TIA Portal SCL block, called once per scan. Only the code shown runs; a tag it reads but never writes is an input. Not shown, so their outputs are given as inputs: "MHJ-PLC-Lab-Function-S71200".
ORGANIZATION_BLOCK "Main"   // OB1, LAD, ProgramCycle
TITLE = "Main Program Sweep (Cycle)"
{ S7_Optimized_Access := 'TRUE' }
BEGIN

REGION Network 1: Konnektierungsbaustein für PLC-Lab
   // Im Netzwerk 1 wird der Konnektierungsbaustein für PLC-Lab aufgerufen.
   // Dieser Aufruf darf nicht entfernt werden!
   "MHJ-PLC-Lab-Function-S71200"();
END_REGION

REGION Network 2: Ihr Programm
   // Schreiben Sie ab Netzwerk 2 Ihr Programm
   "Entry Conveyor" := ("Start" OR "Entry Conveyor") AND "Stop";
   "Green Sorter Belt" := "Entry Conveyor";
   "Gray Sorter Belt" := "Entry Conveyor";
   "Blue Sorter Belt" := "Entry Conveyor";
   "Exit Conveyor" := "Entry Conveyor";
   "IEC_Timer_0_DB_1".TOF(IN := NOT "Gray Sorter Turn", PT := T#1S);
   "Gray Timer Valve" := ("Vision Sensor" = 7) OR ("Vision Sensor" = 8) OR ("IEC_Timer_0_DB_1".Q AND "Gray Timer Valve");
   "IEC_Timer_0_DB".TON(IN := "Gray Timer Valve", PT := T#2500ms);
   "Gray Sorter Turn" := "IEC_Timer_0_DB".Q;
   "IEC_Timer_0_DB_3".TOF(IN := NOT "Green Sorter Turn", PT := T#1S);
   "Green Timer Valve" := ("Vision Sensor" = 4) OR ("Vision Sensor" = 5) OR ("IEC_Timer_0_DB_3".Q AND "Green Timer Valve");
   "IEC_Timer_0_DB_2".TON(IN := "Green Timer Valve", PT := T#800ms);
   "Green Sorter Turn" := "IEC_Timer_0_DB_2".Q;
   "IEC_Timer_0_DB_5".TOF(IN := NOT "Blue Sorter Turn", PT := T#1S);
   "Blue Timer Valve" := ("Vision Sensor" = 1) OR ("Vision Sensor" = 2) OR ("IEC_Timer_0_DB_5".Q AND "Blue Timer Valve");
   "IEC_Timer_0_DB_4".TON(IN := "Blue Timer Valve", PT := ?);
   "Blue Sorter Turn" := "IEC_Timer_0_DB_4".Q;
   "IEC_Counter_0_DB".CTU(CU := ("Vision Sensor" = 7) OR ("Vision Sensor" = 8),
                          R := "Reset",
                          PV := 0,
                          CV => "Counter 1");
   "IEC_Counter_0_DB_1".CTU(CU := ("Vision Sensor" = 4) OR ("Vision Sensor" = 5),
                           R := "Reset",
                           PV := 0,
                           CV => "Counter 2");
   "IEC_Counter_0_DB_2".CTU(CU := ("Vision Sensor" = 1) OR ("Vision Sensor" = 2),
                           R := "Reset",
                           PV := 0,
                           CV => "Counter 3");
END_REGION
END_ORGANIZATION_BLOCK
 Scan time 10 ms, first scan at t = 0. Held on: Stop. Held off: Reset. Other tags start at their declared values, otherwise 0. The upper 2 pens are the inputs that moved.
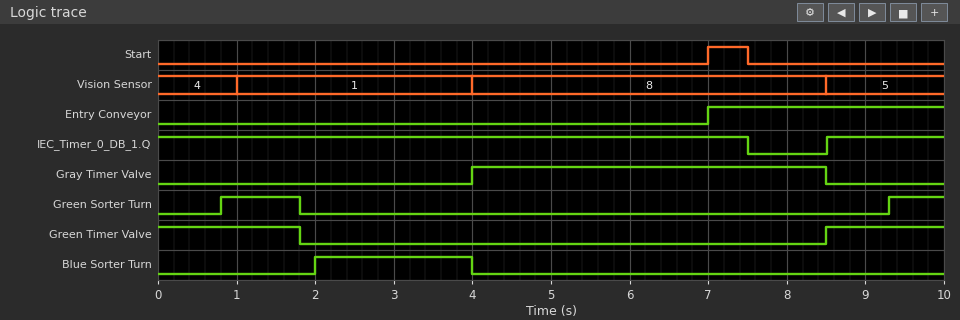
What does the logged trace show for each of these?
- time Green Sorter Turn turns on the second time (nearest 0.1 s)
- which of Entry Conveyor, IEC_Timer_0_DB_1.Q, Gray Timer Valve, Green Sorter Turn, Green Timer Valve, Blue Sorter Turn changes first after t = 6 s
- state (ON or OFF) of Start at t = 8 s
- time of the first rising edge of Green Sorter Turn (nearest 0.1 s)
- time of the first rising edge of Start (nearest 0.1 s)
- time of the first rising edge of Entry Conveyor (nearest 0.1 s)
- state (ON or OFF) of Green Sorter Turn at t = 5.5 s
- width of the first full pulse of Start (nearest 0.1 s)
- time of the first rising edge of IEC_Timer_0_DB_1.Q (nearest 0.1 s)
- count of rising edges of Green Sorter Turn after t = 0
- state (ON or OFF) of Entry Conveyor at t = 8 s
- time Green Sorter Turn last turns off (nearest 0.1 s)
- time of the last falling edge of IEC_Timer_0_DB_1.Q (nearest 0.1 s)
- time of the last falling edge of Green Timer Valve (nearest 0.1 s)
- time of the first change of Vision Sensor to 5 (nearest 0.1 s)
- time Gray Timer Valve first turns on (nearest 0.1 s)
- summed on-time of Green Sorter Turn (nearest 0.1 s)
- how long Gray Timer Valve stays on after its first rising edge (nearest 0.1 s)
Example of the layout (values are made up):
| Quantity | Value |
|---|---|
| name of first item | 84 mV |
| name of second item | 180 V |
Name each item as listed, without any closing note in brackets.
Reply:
| Quantity | Value |
|---|---|
| time Green Sorter Turn turns on the second time | 9.3 s |
| which of Entry Conveyor, IEC_Timer_0_DB_1.Q, Gray Timer Valve, Green Sorter Turn, Green Timer Valve, Blue Sorter Turn changes first after t = 6 s | Entry Conveyor |
| state (ON or OFF) of Start at t = 8 s | OFF |
| time of the first rising edge of Green Sorter Turn | 0.8 s |
| time of the first rising edge of Start | 7.0 s |
| time of the first rising edge of Entry Conveyor | 7.0 s |
| state (ON or OFF) of Green Sorter Turn at t = 5.5 s | OFF |
| width of the first full pulse of Start | 0.5 s |
| time of the first rising edge of IEC_Timer_0_DB_1.Q | 8.5 s |
| count of rising edges of Green Sorter Turn after t = 0 | 2 |
| state (ON or OFF) of Entry Conveyor at t = 8 s | ON |
| time Green Sorter Turn last turns off | 1.8 s |
| time of the last falling edge of IEC_Timer_0_DB_1.Q | 7.5 s |
| time of the last falling edge of Green Timer Valve | 1.8 s |
| time of the first change of Vision Sensor to 5 | 8.5 s |
| time Gray Timer Valve first turns on | 4.0 s |
| summed on-time of Green Sorter Turn | 1.7 s |
| how long Gray Timer Valve stays on after its first rising edge | 4.5 s |
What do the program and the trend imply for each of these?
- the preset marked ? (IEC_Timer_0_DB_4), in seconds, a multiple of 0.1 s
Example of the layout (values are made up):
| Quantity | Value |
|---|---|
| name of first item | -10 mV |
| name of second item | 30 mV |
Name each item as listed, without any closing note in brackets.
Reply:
| Quantity | Value |
|---|---|
| the preset marked ? (IEC_Timer_0_DB_4), in seconds, a multiple of 0.1 s | 1.0 s |
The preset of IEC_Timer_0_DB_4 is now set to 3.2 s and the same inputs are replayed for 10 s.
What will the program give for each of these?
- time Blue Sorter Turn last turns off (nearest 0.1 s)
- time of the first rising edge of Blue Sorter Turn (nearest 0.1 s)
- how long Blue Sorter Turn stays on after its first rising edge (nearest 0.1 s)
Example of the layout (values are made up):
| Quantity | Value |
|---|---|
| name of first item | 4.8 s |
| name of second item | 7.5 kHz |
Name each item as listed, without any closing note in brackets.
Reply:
| Quantity | Value |
|---|---|
| time Blue Sorter Turn last turns off | 5.2 s |
| time of the first rising edge of Blue Sorter Turn | 4.2 s |
| how long Blue Sorter Turn stays on after its first rising edge | 1.0 s |
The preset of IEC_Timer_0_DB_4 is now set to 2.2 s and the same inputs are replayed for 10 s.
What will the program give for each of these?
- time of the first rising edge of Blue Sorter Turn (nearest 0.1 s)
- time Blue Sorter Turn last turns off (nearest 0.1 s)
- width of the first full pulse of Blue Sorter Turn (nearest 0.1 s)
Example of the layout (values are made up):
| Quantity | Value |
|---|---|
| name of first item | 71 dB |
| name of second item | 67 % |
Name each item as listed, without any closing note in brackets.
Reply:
| Quantity | Value |
|---|---|
| time of the first rising edge of Blue Sorter Turn | 3.2 s |
| time Blue Sorter Turn last turns off | 4.2 s |
| width of the first full pulse of Blue Sorter Turn | 1.0 s |
